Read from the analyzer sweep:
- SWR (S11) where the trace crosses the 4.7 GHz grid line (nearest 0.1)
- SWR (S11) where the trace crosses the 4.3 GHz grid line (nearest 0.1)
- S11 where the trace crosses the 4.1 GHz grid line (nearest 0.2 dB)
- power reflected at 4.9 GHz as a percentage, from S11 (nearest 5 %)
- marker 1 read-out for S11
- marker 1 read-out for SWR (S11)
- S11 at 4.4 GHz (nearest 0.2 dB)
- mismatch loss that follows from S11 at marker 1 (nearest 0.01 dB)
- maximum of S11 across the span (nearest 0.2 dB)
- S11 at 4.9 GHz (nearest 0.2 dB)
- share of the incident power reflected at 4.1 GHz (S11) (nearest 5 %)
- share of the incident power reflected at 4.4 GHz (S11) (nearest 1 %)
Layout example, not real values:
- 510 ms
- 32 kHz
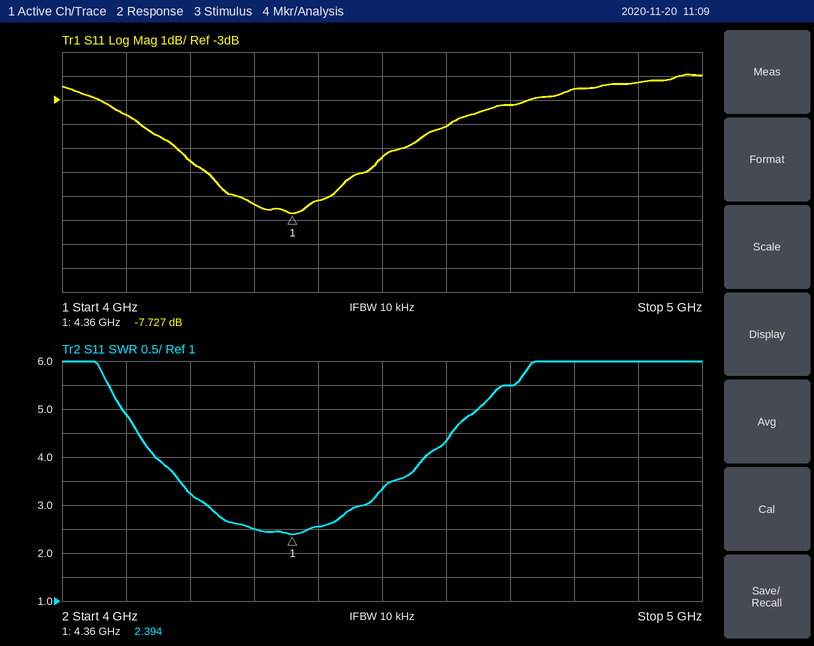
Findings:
- 5.5
- 2.5
- -3.6 dB
- 60 %
- -7.727 dB
- 2.394
- -7.2 dB
- 0.80 dB
- -2.0 dB
- -2.2 dB
- 45 %
- 19 %
